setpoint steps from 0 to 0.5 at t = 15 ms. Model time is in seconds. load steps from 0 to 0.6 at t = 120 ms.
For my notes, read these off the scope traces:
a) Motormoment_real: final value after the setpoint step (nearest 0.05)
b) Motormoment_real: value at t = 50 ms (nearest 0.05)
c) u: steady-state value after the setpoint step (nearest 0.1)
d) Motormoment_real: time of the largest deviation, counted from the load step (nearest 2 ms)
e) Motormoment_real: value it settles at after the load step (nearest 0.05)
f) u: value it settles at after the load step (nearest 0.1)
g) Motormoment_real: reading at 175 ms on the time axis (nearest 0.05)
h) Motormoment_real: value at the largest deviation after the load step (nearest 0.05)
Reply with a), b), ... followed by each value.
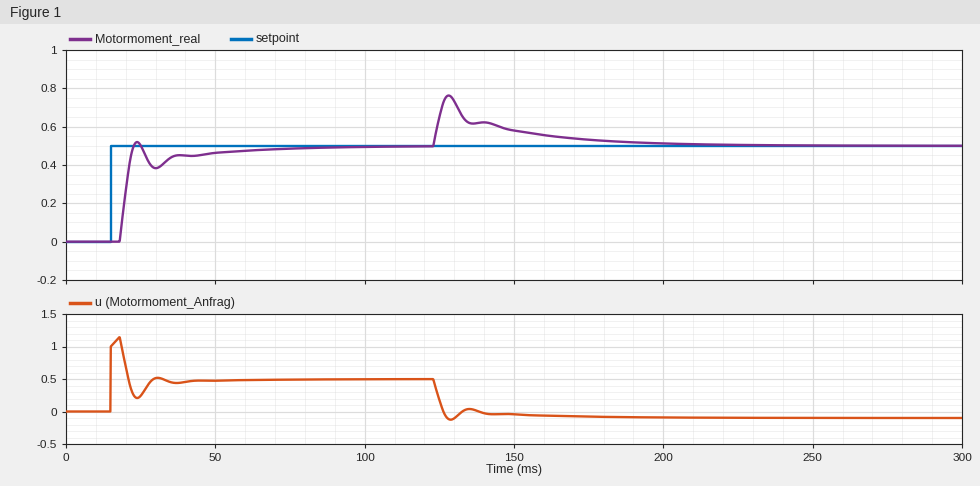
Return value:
a) 0.50
b) 0.45
c) 0.5
d) 8 ms
e) 0.50
f) -0.1
g) 0.55
h) 0.75
